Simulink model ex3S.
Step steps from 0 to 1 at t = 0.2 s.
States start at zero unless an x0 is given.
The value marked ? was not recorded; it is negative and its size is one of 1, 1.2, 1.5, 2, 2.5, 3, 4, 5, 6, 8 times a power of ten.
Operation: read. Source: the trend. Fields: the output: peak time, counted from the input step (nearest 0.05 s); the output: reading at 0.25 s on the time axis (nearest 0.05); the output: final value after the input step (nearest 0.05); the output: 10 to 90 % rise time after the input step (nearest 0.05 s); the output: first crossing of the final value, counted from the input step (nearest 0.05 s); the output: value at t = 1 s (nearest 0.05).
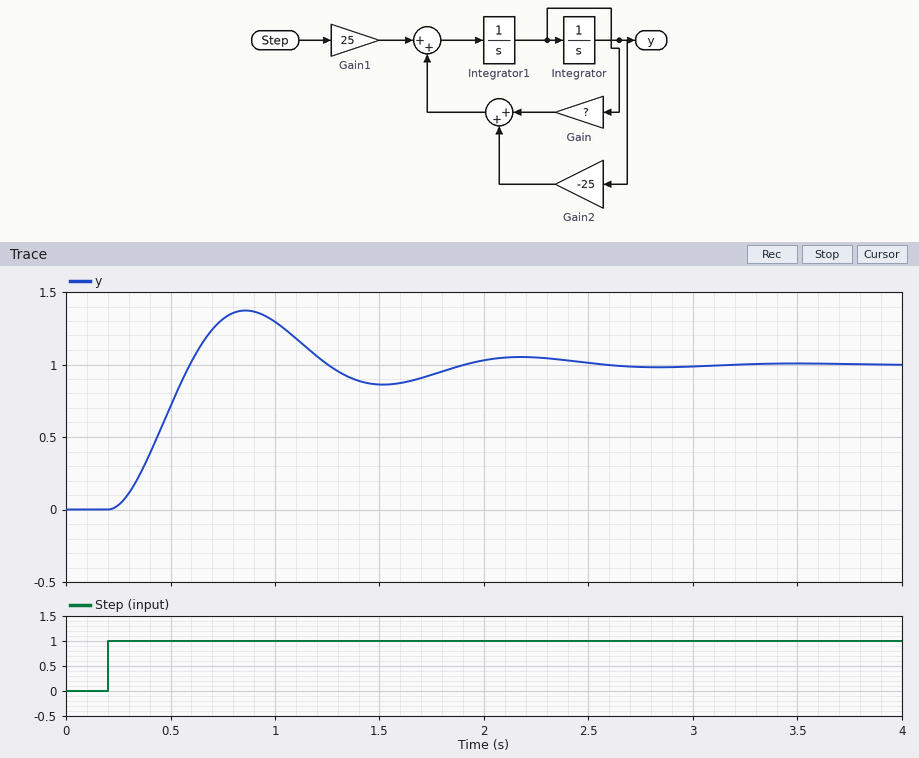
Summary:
0.65 s
0.05
1.00
0.25 s
0.40 s
1.30
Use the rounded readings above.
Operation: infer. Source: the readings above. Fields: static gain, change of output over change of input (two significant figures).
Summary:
1.0
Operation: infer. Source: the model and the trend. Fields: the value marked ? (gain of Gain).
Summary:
-3
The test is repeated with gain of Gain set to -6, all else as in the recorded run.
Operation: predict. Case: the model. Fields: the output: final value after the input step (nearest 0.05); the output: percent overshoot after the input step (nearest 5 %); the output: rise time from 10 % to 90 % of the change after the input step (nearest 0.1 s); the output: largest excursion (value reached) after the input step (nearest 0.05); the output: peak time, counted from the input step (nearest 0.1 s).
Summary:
1.00
10 %
0.4 s
1.10
0.8 s
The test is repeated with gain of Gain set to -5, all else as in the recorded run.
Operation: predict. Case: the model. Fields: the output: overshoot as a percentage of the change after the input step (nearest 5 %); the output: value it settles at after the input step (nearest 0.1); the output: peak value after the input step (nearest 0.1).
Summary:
15 %
1.0
1.2
